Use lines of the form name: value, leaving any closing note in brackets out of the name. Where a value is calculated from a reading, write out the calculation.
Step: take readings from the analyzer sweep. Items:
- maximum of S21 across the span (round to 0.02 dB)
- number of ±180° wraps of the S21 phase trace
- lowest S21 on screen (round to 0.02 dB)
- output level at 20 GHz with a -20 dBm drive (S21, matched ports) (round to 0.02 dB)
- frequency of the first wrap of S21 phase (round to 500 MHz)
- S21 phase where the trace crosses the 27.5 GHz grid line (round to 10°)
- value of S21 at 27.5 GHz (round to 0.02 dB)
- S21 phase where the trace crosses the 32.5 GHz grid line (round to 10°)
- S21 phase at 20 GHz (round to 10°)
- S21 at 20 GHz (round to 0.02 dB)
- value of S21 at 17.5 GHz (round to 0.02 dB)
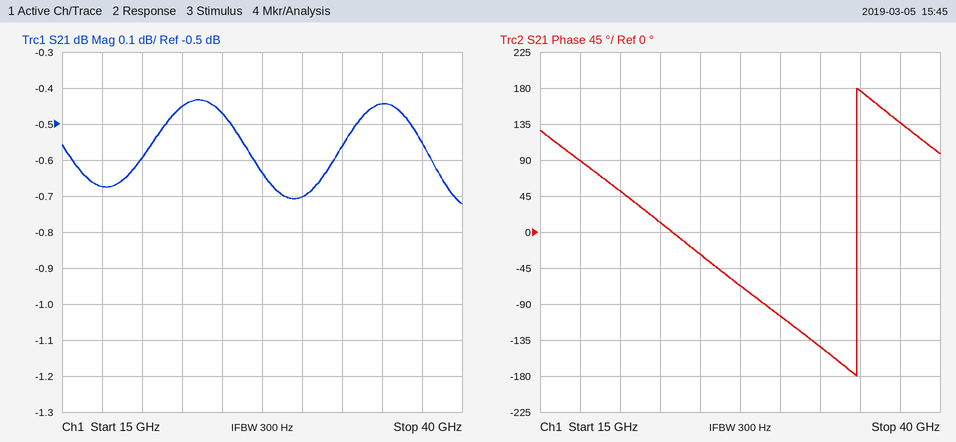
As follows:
maximum of S21 across the span: -0.44 dB
number of ±180° wraps of the S21 phase trace: 1
lowest S21 on screen: -0.72 dB
output level at 20 GHz with a -20 dBm drive (S21, matched ports): -20 dBm + (-0.60 dB) = -20.60 dBm
frequency of the first wrap of S21 phase: 35.0 GHz
S21 phase where the trace crosses the 27.5 GHz grid line: -70°
value of S21 at 27.5 GHz: -0.64 dB
S21 phase where the trace crosses the 32.5 GHz grid line: -140°
S21 phase at 20 GHz: 50°
S21 at 20 GHz: -0.60 dB
value of S21 at 17.5 GHz: -0.68 dB
